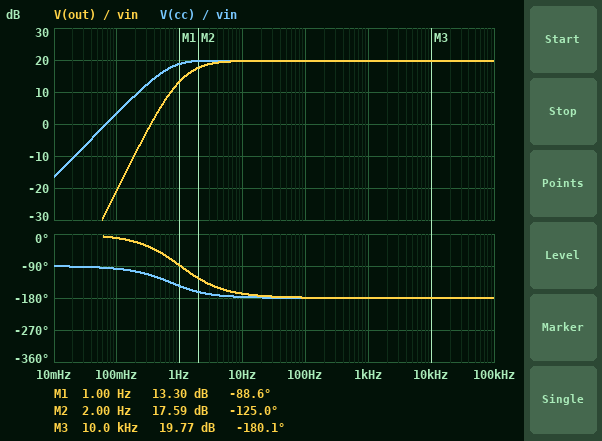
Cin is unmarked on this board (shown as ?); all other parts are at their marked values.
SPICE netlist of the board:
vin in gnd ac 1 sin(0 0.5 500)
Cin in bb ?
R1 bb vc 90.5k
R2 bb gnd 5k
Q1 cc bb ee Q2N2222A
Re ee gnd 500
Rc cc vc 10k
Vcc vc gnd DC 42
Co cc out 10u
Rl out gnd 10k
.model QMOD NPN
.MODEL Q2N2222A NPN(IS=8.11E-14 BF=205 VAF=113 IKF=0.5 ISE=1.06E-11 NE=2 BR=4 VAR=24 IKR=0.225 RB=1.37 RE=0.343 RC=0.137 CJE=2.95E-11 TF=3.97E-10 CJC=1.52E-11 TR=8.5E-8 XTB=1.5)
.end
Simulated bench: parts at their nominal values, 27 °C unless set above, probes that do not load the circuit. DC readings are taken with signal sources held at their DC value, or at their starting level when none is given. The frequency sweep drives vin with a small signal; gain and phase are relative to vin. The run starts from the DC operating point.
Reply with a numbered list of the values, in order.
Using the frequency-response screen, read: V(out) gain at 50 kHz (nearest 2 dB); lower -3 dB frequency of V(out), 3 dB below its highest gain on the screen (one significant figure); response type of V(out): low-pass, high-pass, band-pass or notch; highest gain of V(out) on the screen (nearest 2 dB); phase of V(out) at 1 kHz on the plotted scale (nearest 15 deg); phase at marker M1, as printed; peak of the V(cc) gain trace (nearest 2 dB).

1. 20 dB
2. 2 Hz
3. high-pass
4. 20 dB
5. -180 deg
6. -88.6 deg
7. 20 dB
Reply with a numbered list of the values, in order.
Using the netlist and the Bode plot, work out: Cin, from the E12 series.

1. 27 µF
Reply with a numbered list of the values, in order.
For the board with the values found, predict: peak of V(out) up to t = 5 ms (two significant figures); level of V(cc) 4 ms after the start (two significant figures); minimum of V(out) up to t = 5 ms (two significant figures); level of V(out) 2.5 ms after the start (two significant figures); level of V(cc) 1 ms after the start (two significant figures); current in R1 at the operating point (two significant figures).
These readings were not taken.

1. 4.9 V
2. 12 V
3. -4.9 V
4. -4.9 V
5. 12 V
6. 440 µA
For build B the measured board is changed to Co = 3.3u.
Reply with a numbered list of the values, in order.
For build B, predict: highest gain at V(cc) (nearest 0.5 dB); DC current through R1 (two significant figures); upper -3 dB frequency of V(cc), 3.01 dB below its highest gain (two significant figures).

1. 22.5 dB
2. 440 µA
3. 860 kHz
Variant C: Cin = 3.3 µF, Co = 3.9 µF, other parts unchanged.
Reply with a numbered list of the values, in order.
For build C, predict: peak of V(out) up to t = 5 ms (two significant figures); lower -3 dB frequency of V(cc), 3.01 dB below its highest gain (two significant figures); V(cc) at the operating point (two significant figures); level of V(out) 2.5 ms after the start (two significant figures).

1. 5.0 V
2. 9.5 Hz
3. 12 V
4. -4.8 V
